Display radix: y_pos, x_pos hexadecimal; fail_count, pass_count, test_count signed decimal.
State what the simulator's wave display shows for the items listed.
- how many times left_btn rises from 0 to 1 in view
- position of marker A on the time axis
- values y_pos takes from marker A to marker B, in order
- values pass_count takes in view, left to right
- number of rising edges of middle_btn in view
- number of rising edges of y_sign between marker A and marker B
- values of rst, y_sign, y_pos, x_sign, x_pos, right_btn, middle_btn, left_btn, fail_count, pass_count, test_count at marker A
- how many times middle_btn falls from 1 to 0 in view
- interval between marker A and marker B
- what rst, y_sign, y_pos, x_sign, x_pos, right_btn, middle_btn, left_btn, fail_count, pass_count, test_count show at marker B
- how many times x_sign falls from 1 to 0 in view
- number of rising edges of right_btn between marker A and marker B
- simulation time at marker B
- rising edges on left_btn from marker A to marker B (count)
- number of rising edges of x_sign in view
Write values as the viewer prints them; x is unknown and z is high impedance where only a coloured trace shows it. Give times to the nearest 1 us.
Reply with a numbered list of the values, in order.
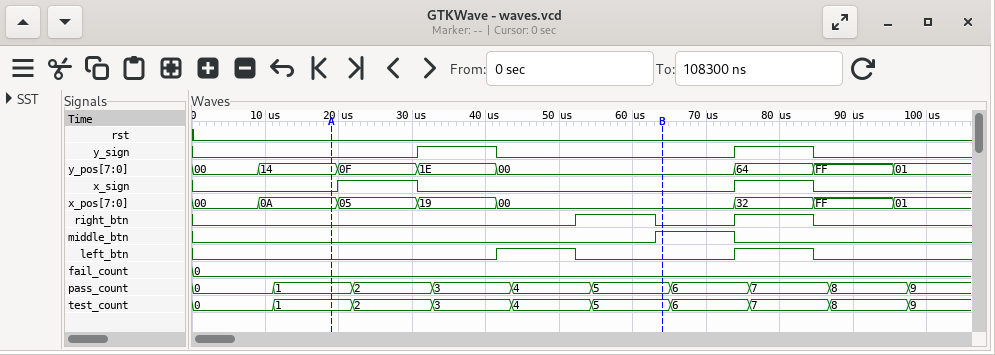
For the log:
1. 2
2. 19 us
3. 14, 0F, 1E, 00
4. 0, 1, 2, 3, 4, 5, 6, 7, 8, 9
5. 1
6. 1
7. rst=0, y_sign=0, y_pos=14, x_sign=0, x_pos=0A, right_btn=0, middle_btn=0, left_btn=0, fail_count=0, pass_count=1, test_count=1
8. 1
9. 45 us
10. rst=0, y_sign=0, y_pos=00, x_sign=0, x_pos=00, right_btn=0, middle_btn=1, left_btn=0, fail_count=0, pass_count=5, test_count=5
11. 2
12. 1
13. 64 us
14. 1
15. 2
